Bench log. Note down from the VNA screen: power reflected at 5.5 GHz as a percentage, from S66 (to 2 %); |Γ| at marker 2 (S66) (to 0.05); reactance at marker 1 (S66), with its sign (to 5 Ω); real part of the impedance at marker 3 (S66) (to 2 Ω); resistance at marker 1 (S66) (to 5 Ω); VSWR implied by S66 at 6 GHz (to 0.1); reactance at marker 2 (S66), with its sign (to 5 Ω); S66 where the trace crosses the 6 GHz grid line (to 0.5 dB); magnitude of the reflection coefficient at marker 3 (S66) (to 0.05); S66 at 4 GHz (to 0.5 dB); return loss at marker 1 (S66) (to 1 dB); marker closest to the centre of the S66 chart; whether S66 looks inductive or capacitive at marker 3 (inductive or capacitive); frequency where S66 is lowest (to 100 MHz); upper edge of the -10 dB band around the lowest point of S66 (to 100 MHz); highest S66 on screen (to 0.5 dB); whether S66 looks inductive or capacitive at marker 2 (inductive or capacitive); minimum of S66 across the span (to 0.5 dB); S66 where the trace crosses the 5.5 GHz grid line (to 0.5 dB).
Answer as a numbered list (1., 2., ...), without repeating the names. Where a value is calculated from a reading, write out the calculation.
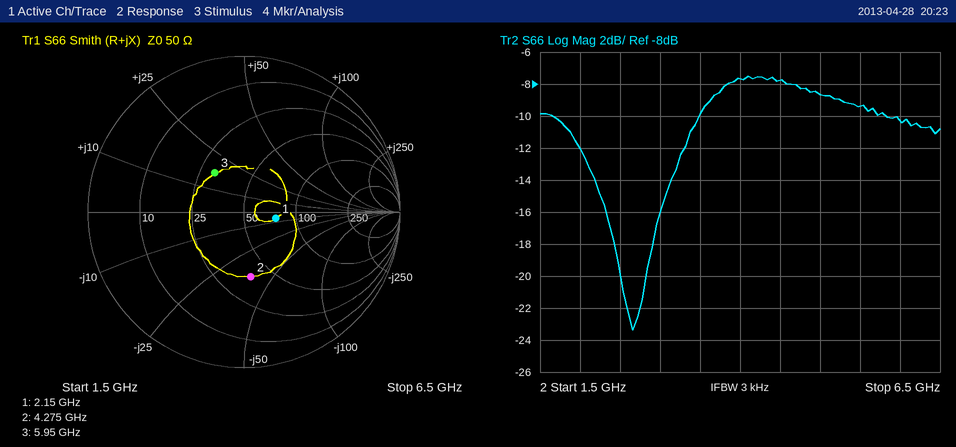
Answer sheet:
1. 10^(-9.5/10) ≈ 11.2 %, so 12 % to the nearest 2 %
2. 0.40
3. -5 Ω
4. 30 Ω
5. 75 Ω
6. |Γ| = 10^(-10.5/20) = 0.2985; VSWR = (1 + 0.2985)/(1 − 0.2985) ≈ 1.9
7. -40 Ω
8. -10.5 dB
9. 0.30
10. -7.5 dB
11. 14 dB
12. marker 1
13. inductive
14. 2.7 GHz
15. 3.5 GHz
16. -7.5 dB
17. capacitive
18. -23.5 dB
19. -9.5 dB
